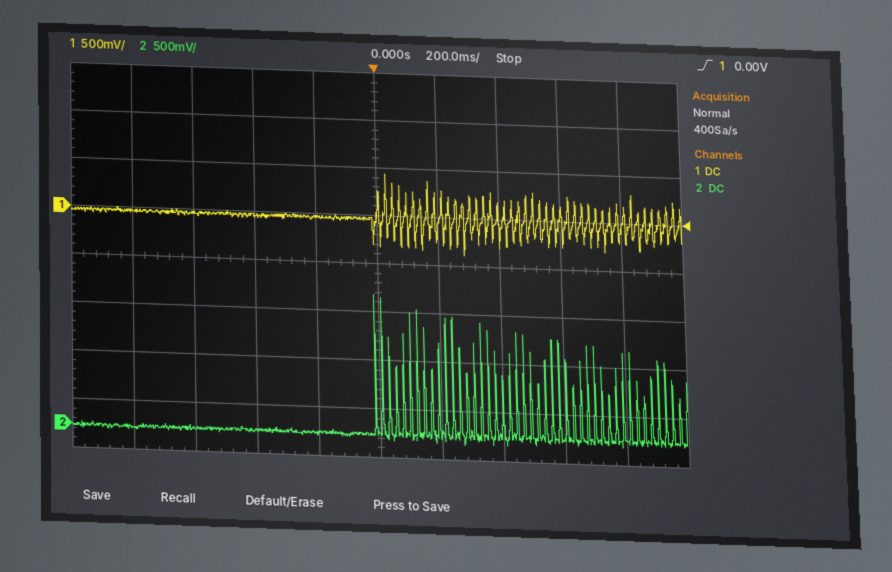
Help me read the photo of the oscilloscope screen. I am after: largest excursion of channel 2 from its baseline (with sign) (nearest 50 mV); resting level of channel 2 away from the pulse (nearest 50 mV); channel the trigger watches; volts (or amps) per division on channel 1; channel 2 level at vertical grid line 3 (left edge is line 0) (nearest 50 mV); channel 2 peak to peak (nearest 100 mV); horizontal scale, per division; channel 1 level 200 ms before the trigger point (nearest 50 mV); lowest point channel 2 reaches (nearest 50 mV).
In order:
+1.45 V
0 mV
channel 1
500 mV
0 mV
1.50 V
200 ms
-50 mV
-100 mV
